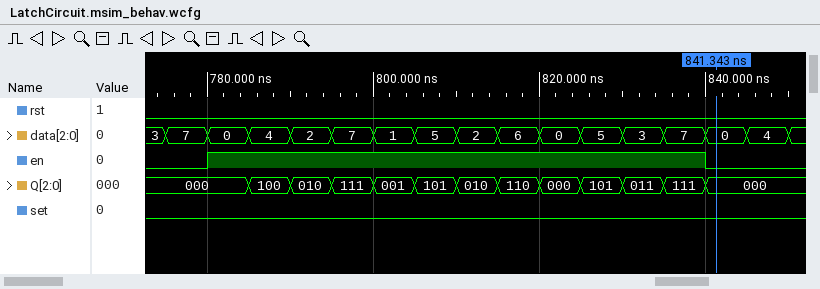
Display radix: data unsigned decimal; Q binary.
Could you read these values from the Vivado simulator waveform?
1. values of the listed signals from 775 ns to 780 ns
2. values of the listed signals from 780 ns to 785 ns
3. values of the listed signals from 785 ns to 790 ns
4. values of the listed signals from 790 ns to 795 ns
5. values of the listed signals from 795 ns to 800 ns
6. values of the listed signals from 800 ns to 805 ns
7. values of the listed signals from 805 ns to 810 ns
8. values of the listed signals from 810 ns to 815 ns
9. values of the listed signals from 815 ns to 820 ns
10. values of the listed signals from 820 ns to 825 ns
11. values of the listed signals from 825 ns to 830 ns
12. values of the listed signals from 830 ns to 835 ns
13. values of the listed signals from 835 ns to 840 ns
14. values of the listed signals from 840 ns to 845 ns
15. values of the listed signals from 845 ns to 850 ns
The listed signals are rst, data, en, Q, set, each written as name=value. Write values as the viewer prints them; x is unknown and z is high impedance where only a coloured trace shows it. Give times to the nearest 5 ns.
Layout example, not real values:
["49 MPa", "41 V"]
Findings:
["rst=0, data=7, en=0, Q=000, set=0", "rst=0, data=0, en=1, Q=000, set=0", "rst=0, data=4, en=1, Q=100, set=0", "rst=0, data=2, en=1, Q=010, set=0", "rst=0, data=7, en=1, Q=111, set=0", "rst=0, data=1, en=1, Q=001, set=0", "rst=0, data=5, en=1, Q=101, set=0", "rst=0, data=2, en=1, Q=010, set=0", "rst=0, data=6, en=1, Q=110, set=0", "rst=0, data=0, en=1, Q=000, set=0", "rst=0, data=5, en=1, Q=101, set=0", "rst=0, data=3, en=1, Q=011, set=0", "rst=0, data=7, en=1, Q=111, set=0", "rst=0, data=0, en=0, Q=000, set=0", "rst=0, data=4, en=0, Q=000, set=0"]
